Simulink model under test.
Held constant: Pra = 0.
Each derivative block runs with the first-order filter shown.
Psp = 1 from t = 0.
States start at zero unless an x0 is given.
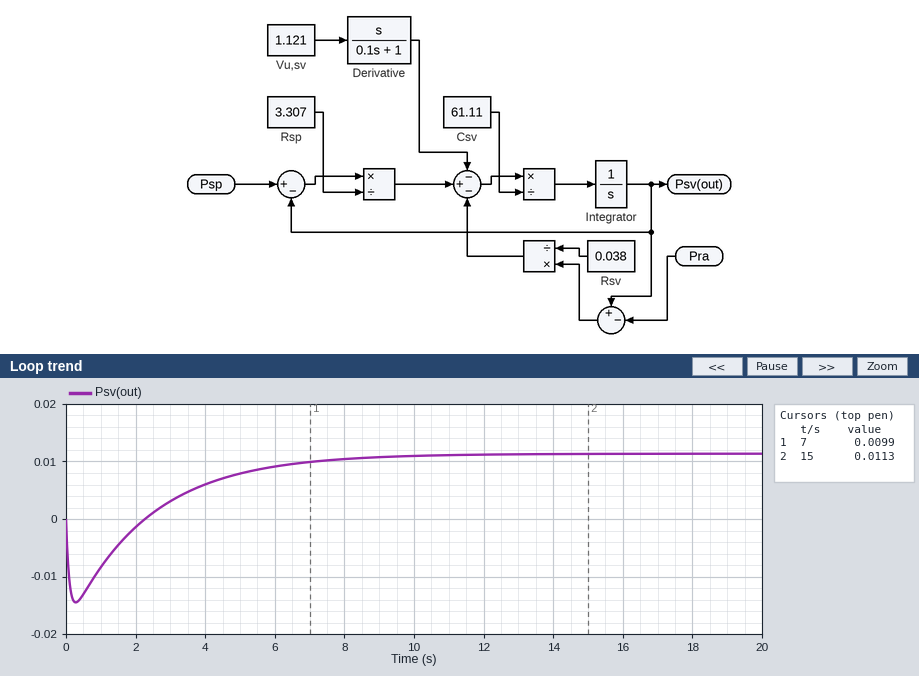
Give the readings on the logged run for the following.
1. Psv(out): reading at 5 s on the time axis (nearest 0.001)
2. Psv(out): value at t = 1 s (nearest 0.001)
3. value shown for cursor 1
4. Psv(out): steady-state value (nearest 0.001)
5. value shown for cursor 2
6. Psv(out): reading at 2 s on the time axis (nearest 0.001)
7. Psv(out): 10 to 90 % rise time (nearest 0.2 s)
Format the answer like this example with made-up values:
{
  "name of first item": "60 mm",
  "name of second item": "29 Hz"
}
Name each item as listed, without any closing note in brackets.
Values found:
{
  "Psv(out): reading at 5 s on the time axis": "0.008",
  "Psv(out): value at t = 1 s": "-0.008",
  "value shown for cursor 1": "0.0099",
  "Psv(out): steady-state value": "0.011",
  "value shown for cursor 2": "0.0113",
  "Psv(out): reading at 2 s on the time axis": "-0.001",
  "Psv(out): 10 to 90 % rise time": "5.0 s"
}
